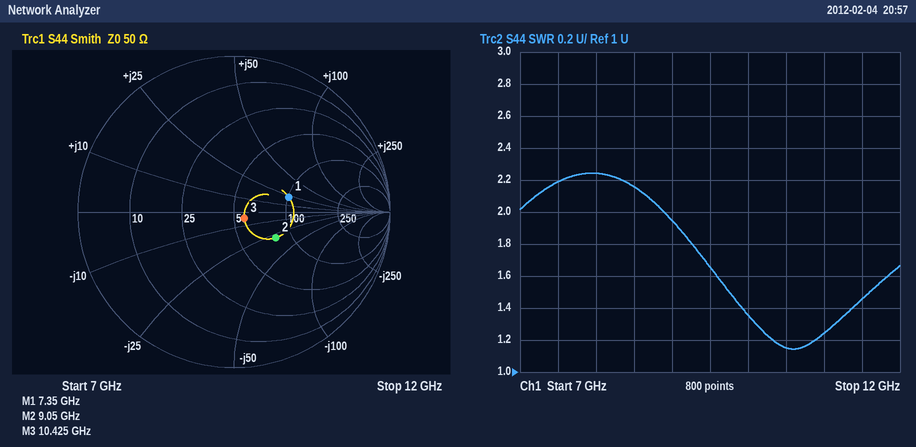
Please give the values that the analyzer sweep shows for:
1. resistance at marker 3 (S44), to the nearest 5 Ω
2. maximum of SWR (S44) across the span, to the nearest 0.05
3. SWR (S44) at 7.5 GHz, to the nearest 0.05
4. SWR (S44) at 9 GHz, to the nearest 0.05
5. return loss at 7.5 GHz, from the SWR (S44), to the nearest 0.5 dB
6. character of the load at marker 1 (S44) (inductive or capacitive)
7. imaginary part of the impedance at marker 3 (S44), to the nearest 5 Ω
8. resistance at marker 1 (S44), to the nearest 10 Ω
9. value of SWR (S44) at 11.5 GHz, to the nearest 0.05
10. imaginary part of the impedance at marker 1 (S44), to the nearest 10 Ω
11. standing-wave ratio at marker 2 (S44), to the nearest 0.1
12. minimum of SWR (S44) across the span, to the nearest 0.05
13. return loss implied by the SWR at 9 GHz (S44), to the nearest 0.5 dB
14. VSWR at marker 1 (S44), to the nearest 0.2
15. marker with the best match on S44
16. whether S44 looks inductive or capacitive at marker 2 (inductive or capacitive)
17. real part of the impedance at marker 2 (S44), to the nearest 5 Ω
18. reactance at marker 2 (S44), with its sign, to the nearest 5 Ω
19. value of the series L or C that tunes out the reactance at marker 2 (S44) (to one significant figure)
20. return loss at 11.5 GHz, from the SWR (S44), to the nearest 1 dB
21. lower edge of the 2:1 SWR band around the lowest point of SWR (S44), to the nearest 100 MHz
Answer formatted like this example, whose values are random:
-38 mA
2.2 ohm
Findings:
55 Ω
2.25
2.20
1.95
8.5 dB
inductive
-5 Ω
100 Ω
1.45
+20 Ω
1.9
1.15
10.0 dB
2.2
marker 3
capacitive
80 Ω
-30 Ω
500 pH
15 dB
8.9 GHz
